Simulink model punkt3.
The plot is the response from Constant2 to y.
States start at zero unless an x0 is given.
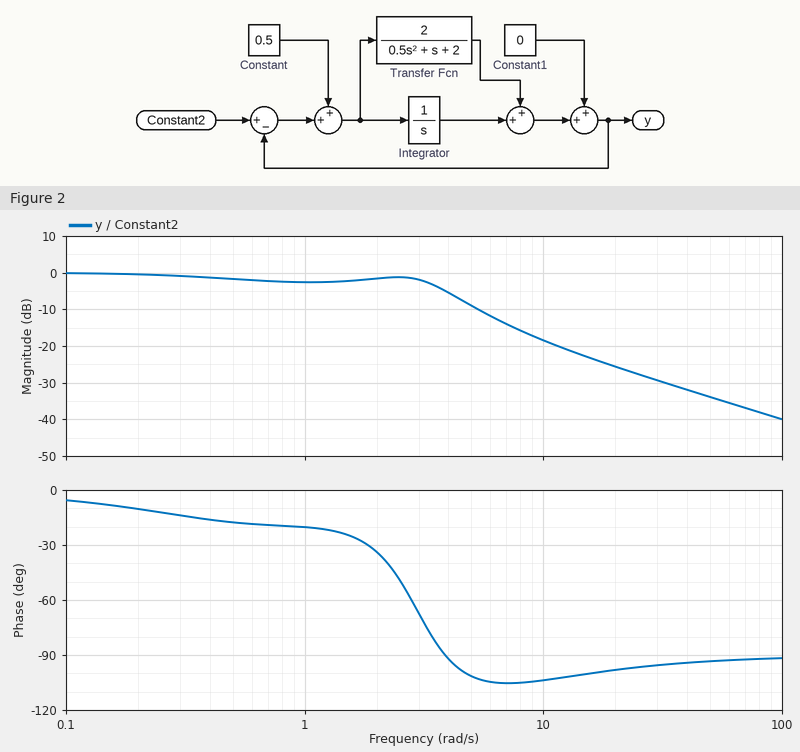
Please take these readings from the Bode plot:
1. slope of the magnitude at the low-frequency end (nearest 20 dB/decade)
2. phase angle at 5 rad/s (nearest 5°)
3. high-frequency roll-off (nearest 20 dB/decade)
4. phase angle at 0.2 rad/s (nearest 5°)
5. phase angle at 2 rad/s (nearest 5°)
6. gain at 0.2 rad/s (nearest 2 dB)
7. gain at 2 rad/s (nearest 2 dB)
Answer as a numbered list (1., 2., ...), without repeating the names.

1. 0 dB/decade
2. -100°
3. -20 dB/decade
4. -10°
5. -35°
6. 0 dB
7. -2 dB
